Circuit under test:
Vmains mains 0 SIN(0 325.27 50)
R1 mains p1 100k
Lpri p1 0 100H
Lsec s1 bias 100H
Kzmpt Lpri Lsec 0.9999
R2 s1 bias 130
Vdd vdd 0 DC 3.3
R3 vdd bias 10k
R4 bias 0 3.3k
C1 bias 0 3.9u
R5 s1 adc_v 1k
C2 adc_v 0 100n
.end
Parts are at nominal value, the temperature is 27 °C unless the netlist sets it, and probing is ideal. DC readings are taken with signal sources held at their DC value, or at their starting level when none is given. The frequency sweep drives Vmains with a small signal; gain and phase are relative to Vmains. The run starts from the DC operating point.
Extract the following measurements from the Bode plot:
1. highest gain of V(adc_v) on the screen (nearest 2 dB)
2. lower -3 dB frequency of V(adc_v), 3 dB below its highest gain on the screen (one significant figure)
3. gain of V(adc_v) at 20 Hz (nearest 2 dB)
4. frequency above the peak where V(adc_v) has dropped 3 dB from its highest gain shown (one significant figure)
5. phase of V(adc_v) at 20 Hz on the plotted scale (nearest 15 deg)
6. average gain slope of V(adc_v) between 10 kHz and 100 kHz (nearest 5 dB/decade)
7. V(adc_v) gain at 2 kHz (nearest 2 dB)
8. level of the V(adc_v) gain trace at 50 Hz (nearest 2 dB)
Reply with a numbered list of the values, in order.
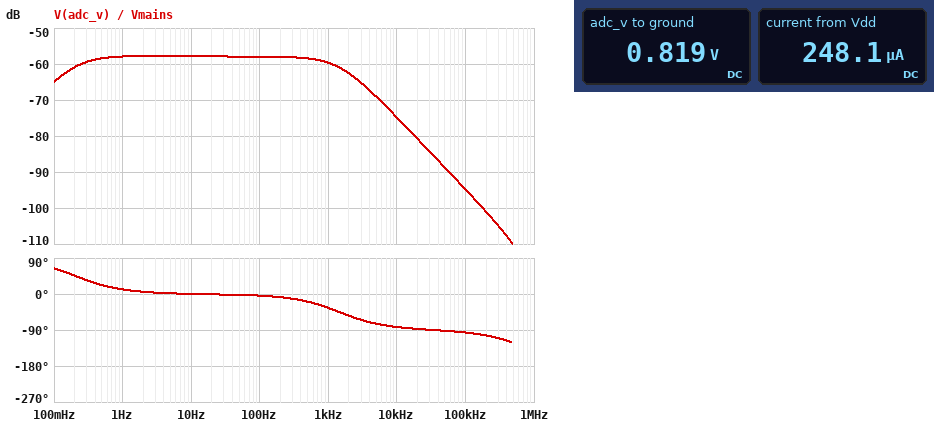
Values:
1. -58 dB
2. 200 mHz
3. -58 dB
4. 1 kHz
5. 0 deg
6. -20 dB/decade
7. -62 dB
8. -58 dB
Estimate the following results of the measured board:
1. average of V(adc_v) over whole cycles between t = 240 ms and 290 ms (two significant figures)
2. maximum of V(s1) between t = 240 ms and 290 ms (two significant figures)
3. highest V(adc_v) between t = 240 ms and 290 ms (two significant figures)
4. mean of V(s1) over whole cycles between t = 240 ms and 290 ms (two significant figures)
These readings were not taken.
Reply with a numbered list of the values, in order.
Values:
1. 820 mV
2. 1.2 V
3. 1.2 V
4. 820 mV
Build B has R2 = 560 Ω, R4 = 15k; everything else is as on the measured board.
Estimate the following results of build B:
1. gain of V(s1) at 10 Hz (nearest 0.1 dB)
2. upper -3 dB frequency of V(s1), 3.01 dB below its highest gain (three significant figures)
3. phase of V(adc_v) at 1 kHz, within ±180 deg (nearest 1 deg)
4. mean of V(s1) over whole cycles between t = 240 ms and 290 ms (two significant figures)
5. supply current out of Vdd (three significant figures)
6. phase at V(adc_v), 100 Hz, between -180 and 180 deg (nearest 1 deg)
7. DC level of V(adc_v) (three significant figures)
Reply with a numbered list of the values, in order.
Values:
1. -45.3 dB
2. 2.78 kHz
3. -44 deg
4. 2.0 V
5. 132 µA
6. -5 deg
7. 1.98 V
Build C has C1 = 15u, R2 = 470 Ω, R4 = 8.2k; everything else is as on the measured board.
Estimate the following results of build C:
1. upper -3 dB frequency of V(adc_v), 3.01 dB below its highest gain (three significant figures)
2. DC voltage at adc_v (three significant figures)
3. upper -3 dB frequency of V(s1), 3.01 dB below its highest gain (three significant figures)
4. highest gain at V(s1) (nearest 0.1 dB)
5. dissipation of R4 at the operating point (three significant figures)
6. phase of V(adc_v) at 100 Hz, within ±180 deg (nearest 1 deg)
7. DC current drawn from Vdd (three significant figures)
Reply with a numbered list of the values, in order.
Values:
1. 1.09 kHz
2. 1.49 V
3. 4.50 kHz
4. -46.7 dB
5. 270 µW
6. -5 deg
7. 181 µA
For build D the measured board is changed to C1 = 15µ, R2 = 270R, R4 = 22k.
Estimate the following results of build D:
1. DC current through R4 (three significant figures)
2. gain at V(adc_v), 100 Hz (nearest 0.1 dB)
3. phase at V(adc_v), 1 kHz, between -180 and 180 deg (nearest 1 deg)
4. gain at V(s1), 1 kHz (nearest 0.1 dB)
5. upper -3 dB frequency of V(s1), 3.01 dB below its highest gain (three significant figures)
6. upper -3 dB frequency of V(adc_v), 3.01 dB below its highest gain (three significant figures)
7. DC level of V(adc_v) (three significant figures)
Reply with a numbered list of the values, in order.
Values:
1. 103 µA
2. -51.5 dB
3. -38 deg
4. -52.1 dB
5. 405 kHz
6. 1.26 kHz
7. 2.27 V
